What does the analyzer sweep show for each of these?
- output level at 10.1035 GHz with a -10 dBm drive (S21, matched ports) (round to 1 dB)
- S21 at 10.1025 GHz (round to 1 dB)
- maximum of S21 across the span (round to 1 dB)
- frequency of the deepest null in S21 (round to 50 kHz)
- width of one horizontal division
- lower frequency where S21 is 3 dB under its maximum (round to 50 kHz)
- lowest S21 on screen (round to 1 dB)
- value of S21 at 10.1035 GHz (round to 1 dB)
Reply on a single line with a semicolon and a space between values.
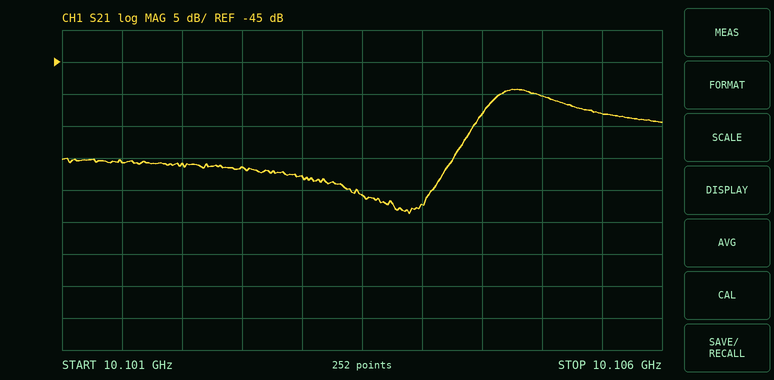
-76 dBm; -61 dB; -49 dB; 10.10390 GHz; 500 kHz; 10.10455 GHz; -69 dB; -66 dB
